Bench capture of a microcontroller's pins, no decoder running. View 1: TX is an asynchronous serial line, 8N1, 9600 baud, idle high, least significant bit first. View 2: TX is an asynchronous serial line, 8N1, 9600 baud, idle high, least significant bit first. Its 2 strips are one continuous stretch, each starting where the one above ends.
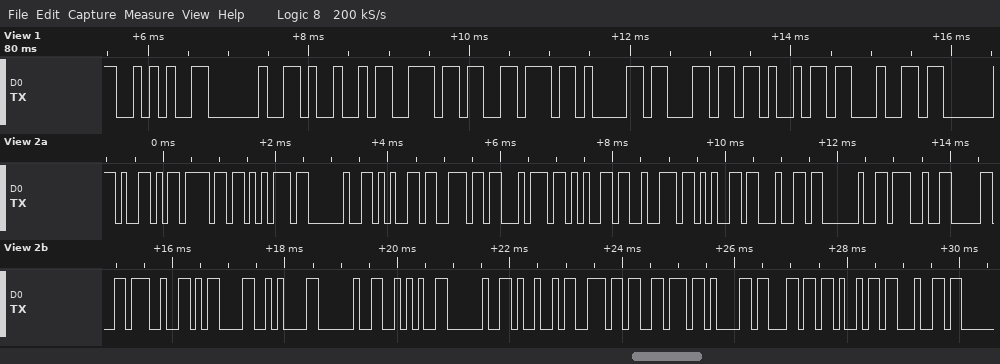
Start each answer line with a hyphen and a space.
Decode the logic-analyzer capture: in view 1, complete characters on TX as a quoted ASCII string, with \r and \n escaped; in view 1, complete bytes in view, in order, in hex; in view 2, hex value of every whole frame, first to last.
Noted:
- "* Invalid"
- 0x2A 0x20 0x49 0x6E 0x76 0x61 0x6C 0x69 0x64
- 59 6F 75 20 65 6E 74 65 72 65 64 20 27 30 27 0D 0A 20 2A 20 49 6E 76 61 6C 69 64
